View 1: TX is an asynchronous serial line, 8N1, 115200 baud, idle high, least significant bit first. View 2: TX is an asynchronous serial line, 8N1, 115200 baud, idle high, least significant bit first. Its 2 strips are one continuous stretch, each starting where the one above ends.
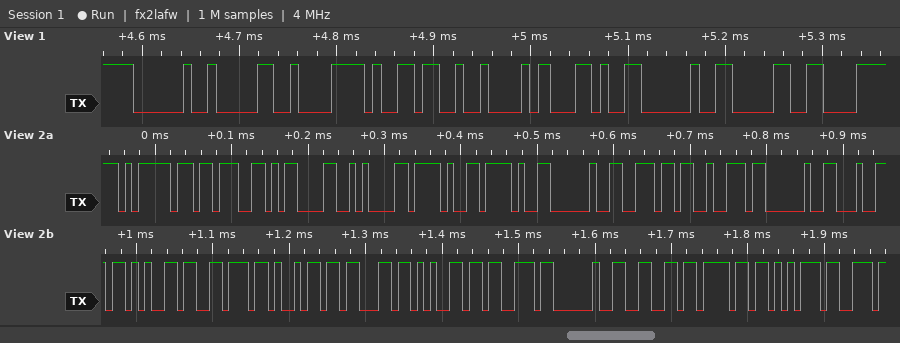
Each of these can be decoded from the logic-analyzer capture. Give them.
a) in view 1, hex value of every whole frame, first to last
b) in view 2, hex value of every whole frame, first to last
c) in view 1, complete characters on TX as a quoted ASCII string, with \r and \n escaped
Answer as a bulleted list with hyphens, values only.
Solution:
- 0x20 0x30 0x78 0x36 0x42 0x2C 0x20 0x30
- 7D 3B 0D 0A 2F 2F 20 6E 72 20 64 65 76 69 63 65 73 20 66 6F 75
- " 0x6B, 0"
